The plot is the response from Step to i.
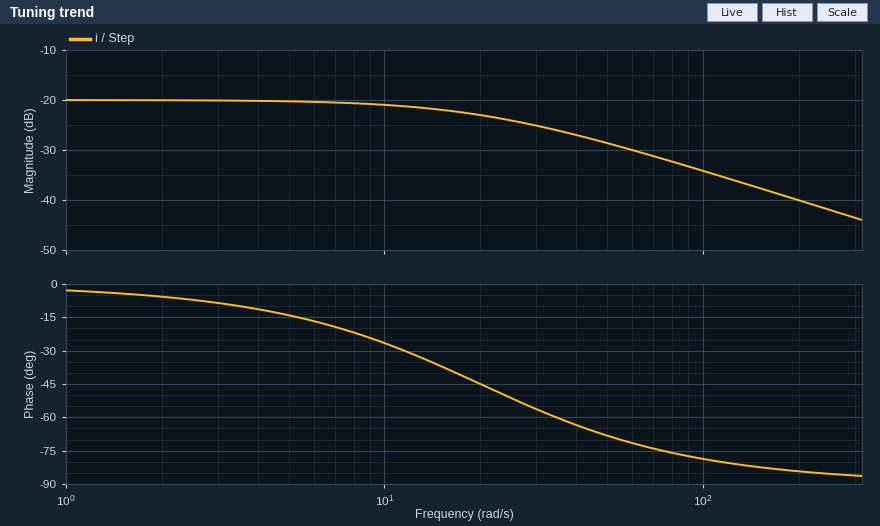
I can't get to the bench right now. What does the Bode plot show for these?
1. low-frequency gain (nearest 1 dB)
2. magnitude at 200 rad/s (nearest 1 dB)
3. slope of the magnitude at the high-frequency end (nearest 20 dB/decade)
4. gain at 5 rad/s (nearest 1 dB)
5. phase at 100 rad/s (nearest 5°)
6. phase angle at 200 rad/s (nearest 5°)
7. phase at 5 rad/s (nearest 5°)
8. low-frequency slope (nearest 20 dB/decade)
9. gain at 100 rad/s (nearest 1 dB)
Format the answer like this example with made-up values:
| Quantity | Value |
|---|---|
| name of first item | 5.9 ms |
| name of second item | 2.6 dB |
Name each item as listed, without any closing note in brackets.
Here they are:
| Quantity | Value |
|---|---|
| low-frequency gain | -20 dB |
| magnitude at 200 rad/s | -40 dB |
| slope of the magnitude at the high-frequency end | -20 dB/decade |
| gain at 5 rad/s | -20 dB |
| phase at 100 rad/s | -80° |
| phase angle at 200 rad/s | -85° |
| phase at 5 rad/s | -15° |
| low-frequency slope | 0 dB/decade |
| gain at 100 rad/s | -34 dB |
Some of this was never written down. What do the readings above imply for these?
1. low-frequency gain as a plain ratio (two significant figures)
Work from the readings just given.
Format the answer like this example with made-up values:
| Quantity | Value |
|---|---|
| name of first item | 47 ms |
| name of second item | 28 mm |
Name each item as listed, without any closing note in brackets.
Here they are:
| Quantity | Value |
|---|---|
| low-frequency gain as a plain ratio | 0.10 |
